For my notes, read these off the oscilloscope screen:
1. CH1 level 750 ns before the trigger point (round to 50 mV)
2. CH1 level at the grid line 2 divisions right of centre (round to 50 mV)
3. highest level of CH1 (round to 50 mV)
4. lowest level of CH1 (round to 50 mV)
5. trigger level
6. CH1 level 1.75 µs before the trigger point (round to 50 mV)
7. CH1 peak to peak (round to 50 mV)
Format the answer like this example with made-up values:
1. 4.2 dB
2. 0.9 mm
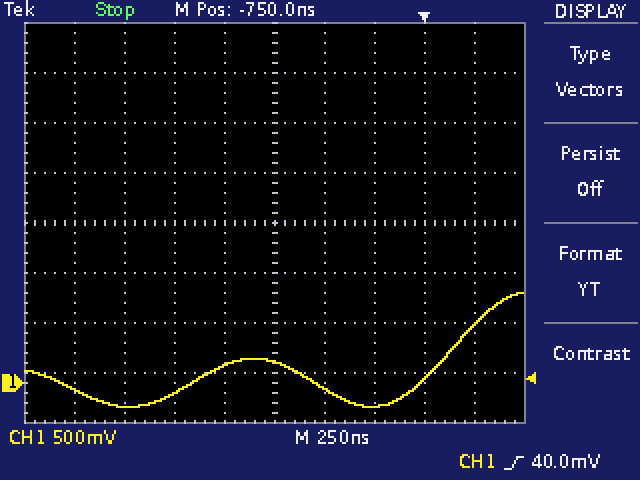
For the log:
1. 200 mV
2. -250 mV
3. 900 mV
4. -250 mV
5. 40.0 mV
6. -50 mV
7. 1.15 V
